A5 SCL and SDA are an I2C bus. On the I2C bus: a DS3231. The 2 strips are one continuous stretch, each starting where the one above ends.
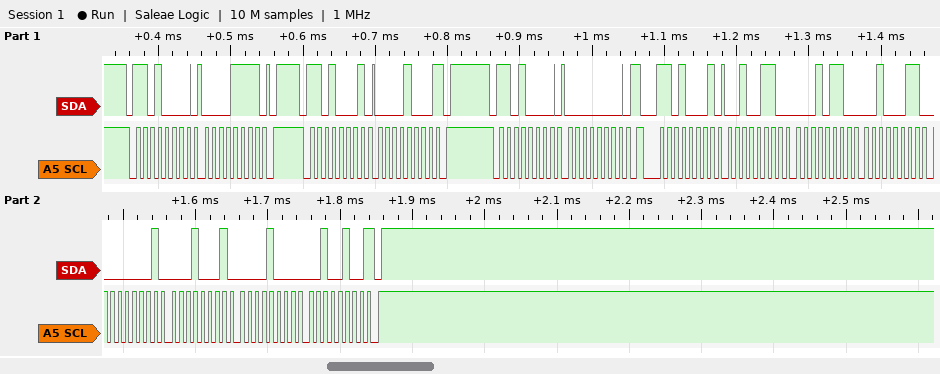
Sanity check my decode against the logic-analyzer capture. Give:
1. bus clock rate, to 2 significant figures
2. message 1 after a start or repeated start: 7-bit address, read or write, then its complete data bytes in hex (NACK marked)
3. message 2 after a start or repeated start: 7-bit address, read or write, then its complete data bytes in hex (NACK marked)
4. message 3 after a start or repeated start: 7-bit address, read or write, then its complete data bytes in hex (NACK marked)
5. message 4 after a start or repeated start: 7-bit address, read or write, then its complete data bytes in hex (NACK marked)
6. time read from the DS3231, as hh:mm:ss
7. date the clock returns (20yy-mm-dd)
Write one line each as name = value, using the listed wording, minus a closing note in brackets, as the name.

bus clock rate, to 2 significant figures = 100 kHz
message 1 after a start or repeated start: 7-bit address, read or write, then its complete data bytes in hex = 0x68 write: 0F
message 2 after a start or repeated start: 7-bit address, read or write, then its complete data bytes in hex = 0x68 read: 08 NACK
message 3 after a start or repeated start: 7-bit address, read or write, then its complete data bytes in hex = 0x68 write: 00
message 4 after a start or repeated start: 7-bit address, read or write, then its complete data bytes in hex = 0x68 read: 26 16 23 01 11 08 24 NACK
time read from the DS3231, as hh:mm:ss = 23:16:26
date the clock returns = 2024-08-11
